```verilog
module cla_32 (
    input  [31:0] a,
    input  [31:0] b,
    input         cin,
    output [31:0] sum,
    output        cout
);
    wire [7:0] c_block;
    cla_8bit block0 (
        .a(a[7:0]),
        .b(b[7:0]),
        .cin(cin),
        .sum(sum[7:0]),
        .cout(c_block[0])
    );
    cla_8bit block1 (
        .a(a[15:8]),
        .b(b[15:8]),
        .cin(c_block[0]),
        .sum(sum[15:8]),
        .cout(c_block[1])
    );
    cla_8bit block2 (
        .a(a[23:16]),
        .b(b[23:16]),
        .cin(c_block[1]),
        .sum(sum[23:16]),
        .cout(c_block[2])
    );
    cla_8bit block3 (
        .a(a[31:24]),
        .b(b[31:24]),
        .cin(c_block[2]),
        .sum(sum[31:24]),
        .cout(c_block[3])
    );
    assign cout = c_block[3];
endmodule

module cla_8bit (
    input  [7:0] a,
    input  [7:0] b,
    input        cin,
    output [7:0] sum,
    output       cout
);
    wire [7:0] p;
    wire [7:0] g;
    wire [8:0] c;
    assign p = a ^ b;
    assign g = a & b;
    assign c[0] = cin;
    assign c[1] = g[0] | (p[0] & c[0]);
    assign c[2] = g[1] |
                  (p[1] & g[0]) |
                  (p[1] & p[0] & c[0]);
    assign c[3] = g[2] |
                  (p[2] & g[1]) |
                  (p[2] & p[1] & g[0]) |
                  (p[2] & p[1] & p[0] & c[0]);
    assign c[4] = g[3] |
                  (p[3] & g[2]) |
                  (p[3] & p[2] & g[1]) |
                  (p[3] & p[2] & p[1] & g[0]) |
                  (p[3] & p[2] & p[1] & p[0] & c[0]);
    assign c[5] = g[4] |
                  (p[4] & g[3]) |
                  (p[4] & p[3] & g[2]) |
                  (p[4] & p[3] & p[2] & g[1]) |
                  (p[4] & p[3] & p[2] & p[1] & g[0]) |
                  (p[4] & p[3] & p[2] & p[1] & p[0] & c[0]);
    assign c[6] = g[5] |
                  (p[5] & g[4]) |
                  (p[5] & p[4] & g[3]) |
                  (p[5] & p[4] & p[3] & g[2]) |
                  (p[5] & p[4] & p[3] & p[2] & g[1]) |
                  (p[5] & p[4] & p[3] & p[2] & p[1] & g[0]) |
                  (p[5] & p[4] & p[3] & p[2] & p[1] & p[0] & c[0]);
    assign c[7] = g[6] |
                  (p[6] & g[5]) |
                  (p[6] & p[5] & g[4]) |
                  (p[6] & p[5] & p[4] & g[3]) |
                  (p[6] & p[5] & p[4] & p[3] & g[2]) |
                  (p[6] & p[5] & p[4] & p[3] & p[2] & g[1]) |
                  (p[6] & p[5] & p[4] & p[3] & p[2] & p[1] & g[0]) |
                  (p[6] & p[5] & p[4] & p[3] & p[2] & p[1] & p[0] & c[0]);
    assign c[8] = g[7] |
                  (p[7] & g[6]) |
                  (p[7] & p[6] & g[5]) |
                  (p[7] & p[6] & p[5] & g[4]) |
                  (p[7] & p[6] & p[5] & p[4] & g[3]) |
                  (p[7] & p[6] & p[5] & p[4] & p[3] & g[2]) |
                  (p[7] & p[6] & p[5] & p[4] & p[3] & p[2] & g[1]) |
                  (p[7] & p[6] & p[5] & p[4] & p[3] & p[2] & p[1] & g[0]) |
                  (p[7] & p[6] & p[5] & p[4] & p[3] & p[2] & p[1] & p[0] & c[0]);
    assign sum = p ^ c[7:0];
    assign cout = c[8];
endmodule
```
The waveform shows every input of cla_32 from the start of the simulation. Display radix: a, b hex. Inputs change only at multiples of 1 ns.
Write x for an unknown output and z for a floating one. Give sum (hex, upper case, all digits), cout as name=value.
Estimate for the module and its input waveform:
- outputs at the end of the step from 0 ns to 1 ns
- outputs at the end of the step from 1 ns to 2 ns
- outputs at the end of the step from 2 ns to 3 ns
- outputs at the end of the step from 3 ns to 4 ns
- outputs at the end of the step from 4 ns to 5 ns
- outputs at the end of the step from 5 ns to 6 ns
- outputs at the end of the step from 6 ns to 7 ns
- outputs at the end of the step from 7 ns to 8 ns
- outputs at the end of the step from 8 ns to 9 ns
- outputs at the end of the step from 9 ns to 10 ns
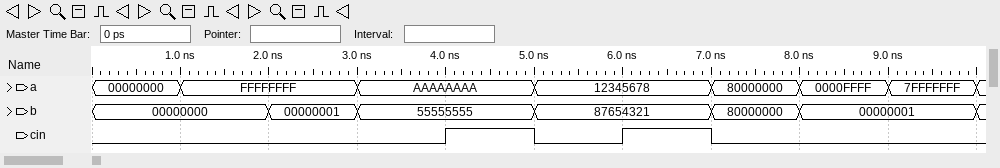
sum=00000000, cout=0
sum=FFFFFFFF, cout=0
sum=00000000, cout=1
sum=FFFFFFFF, cout=0
sum=00000000, cout=1
sum=99999999, cout=0
sum=9999999A, cout=0
sum=00000000, cout=1
sum=00010000, cout=0
sum=80000000, cout=0
